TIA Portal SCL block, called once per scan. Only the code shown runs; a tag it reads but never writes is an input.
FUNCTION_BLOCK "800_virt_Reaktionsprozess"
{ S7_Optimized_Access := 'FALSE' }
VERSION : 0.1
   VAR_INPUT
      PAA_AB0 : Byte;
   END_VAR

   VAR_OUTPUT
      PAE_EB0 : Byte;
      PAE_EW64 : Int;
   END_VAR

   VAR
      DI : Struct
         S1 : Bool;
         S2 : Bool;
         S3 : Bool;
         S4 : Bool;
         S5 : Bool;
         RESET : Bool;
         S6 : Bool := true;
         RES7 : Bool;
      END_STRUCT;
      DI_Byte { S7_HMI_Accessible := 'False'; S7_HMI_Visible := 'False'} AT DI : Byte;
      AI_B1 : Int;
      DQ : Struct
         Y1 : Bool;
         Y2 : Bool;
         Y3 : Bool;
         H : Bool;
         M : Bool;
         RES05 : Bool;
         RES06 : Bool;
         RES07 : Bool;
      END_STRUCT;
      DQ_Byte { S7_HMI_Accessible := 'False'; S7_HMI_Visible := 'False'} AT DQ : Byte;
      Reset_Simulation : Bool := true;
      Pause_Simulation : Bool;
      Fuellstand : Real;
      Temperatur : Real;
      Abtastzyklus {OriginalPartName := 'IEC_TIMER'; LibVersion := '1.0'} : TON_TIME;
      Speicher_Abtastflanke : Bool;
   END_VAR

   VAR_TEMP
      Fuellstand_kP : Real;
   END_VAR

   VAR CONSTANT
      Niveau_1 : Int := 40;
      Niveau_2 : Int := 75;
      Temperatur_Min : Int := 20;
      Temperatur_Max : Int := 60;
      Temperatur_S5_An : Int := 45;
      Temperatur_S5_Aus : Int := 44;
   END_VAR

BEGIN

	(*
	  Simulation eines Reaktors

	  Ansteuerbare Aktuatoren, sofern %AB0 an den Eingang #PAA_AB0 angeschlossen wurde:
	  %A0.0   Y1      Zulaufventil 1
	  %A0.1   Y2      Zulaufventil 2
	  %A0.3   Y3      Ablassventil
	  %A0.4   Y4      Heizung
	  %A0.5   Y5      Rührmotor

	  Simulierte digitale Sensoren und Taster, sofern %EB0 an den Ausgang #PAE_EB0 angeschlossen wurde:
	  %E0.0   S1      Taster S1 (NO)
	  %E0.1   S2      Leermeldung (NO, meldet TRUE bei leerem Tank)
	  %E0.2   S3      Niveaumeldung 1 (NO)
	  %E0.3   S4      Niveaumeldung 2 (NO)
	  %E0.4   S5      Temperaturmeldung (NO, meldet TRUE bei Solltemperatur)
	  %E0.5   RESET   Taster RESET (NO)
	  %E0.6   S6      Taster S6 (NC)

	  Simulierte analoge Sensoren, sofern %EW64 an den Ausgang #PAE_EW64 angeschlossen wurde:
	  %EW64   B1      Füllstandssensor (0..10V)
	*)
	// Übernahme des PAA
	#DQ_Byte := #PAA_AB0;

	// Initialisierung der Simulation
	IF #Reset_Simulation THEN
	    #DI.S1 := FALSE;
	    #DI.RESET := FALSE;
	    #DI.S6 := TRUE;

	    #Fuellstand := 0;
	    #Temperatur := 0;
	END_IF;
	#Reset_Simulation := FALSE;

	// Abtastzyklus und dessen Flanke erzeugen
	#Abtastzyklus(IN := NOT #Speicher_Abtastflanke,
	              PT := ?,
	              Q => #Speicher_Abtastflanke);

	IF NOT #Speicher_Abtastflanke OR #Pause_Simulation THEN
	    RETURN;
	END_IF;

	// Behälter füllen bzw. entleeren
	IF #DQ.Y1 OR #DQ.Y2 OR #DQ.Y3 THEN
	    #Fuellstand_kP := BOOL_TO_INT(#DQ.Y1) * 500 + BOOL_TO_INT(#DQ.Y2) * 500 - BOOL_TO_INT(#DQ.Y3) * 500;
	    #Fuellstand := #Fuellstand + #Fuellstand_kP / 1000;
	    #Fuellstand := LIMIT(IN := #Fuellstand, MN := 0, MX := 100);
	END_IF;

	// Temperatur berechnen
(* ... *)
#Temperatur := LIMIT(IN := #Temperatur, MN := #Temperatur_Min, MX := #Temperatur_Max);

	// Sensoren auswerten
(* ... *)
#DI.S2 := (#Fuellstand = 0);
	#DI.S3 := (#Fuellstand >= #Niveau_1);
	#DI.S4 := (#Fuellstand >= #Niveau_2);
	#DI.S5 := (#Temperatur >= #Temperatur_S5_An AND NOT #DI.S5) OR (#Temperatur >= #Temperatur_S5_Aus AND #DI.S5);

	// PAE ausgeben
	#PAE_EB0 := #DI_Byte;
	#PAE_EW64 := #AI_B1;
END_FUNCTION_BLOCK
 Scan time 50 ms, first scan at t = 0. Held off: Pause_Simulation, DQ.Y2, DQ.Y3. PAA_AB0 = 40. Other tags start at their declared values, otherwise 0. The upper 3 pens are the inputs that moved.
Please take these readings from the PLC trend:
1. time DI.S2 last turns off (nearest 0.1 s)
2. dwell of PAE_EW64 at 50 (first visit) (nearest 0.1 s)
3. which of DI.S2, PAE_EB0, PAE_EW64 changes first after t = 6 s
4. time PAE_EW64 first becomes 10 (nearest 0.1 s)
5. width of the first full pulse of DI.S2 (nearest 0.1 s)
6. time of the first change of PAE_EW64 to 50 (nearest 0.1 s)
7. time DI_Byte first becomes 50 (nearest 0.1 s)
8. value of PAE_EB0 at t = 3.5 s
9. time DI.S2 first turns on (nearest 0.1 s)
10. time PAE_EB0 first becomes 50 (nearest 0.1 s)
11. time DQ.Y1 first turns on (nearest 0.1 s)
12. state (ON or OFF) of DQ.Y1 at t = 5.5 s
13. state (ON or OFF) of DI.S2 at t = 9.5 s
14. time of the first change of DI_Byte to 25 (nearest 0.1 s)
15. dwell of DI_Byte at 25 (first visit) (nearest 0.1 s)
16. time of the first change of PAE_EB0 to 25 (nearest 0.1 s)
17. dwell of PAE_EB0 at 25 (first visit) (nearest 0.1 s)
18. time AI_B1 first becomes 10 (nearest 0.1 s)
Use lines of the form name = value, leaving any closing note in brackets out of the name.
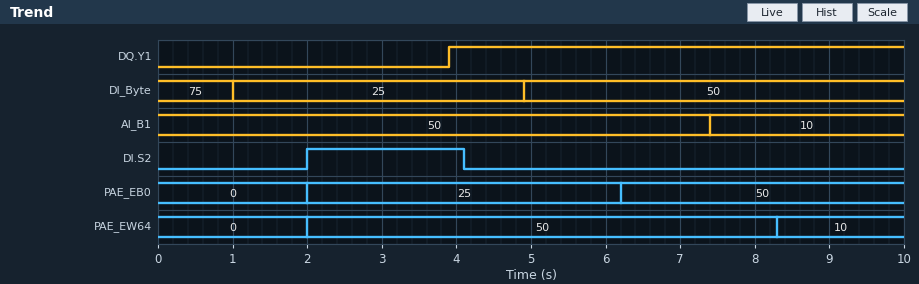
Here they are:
time DI.S2 last turns off = 4.1 s
dwell of PAE_EW64 at 50 (first visit) = 6.3 s
which of DI.S2, PAE_EB0, PAE_EW64 changes first after t = 6 s = PAE_EB0
time PAE_EW64 first becomes 10 = 8.3 s
width of the first full pulse of DI.S2 = 2.1 s
time of the first change of PAE_EW64 to 50 = 2.0 s
time DI_Byte first becomes 50 = 4.9 s
value of PAE_EB0 at t = 3.5 s = 25
time DI.S2 first turns on = 2.0 s
time PAE_EB0 first becomes 50 = 6.2 s
time DQ.Y1 first turns on = 3.9 s
state (ON or OFF) of DQ.Y1 at t = 5.5 s = ON
state (ON or OFF) of DI.S2 at t = 9.5 s = OFF
time of the first change of DI_Byte to 25 = 1.0 s
dwell of DI_Byte at 25 (first visit) = 3.9 s
time of the first change of PAE_EB0 to 25 = 2.0 s
dwell of PAE_EB0 at 25 (first visit) = 4.2 s
time AI_B1 first becomes 10 = 7.4 s
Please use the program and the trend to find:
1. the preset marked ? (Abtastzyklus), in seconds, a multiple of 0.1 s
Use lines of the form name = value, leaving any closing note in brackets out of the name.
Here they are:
the preset marked ? (Abtastzyklus), in seconds, a multiple of 0.1 s = 2.0 s
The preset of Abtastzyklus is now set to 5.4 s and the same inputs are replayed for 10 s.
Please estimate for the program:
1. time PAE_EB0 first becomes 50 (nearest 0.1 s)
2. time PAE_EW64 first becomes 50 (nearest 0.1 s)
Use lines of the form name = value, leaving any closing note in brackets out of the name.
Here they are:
time PAE_EB0 first becomes 50 = 5.4 s
time PAE_EW64 first becomes 50 = 5.4 s
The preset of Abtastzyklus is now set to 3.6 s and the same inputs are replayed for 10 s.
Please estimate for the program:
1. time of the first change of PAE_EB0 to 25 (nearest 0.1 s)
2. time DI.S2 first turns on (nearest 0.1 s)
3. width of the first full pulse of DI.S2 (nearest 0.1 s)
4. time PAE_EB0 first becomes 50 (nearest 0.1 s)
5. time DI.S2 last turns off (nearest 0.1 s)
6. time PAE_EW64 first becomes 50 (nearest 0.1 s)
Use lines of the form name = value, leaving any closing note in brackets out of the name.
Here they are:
time of the first change of PAE_EB0 to 25 = 3.6 s
time DI.S2 first turns on = 3.6 s
width of the first full pulse of DI.S2 = 3.7 s
time PAE_EB0 first becomes 50 = 7.3 s
time DI.S2 last turns off = 7.3 s
time PAE_EW64 first becomes 50 = 3.6 s
